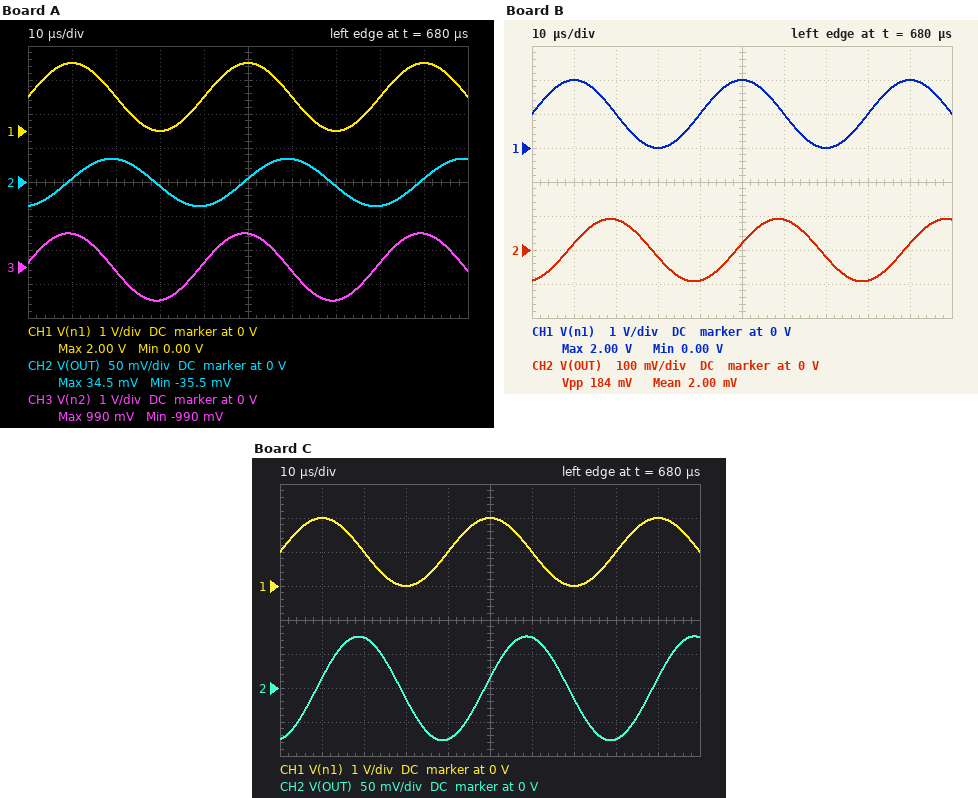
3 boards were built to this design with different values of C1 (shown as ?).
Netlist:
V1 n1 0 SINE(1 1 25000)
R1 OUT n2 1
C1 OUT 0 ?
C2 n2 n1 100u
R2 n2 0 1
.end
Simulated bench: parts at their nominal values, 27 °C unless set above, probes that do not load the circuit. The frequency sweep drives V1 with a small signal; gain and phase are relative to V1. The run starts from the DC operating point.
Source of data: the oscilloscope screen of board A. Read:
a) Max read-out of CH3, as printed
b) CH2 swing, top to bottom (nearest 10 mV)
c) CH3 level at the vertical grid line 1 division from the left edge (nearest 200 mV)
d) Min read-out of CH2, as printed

990 mV
70 mV
1.0 V
-35.5 mV
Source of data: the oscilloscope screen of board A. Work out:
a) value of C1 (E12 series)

180 µF
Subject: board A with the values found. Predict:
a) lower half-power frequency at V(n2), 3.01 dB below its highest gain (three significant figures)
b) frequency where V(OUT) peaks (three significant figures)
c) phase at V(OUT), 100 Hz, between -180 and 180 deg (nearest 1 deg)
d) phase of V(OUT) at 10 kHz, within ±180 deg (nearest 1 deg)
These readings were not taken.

3.51 kHz
1.19 kHz
74 deg
-68 deg
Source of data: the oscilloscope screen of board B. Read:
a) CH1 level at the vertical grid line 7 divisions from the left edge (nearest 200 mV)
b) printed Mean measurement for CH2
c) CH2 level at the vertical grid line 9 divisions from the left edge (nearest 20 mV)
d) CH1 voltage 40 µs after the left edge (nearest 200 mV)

0 V
2.00 mV
20 mV
1.0 V
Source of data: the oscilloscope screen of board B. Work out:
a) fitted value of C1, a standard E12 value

68 µF
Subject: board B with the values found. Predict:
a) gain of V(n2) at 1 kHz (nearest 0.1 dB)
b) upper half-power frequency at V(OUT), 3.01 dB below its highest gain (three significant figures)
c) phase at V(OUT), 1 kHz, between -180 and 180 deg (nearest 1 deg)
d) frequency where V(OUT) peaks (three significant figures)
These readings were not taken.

-7.7 dB
6.13 kHz
26 deg
1.93 kHz
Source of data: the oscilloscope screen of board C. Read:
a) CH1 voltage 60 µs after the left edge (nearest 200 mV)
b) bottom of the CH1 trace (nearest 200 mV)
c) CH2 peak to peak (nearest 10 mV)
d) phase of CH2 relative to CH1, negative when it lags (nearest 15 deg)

1.0 V
0 V
150 mV
-75 deg
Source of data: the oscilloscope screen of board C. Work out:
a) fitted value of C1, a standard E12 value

82 µF
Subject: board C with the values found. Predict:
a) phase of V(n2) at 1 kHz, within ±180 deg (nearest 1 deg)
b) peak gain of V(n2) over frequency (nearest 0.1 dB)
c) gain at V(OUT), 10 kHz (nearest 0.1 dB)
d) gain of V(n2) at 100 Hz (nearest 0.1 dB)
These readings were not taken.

49 deg
0 dB
-15.0 dB
-24.1 dB
